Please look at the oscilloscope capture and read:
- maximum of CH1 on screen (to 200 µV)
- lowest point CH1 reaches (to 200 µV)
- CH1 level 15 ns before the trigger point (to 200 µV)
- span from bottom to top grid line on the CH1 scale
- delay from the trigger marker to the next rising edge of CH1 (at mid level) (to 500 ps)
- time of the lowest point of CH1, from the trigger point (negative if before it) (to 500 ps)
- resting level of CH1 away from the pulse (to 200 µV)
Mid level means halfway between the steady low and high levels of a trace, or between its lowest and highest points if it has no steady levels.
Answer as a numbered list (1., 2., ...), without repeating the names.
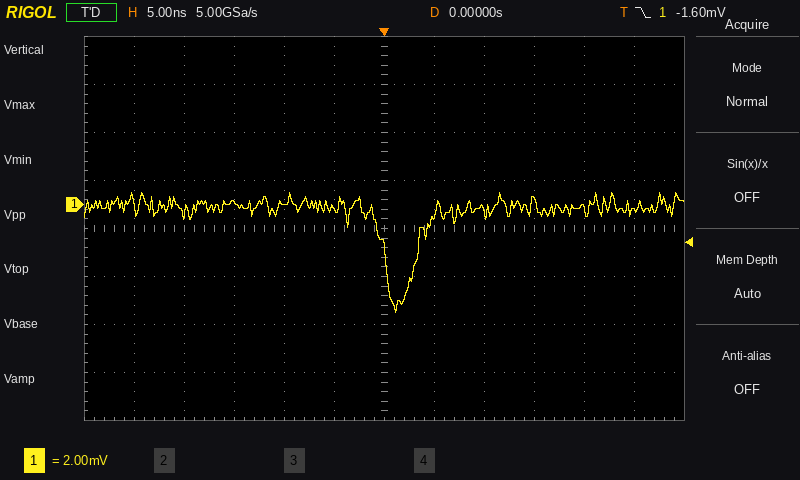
1. 400 µV
2. -4.4 mV
3. 0.0 mV
4. 16 mV
5. 3.5 ns
6. +1.0 ns
7. -200 µV
